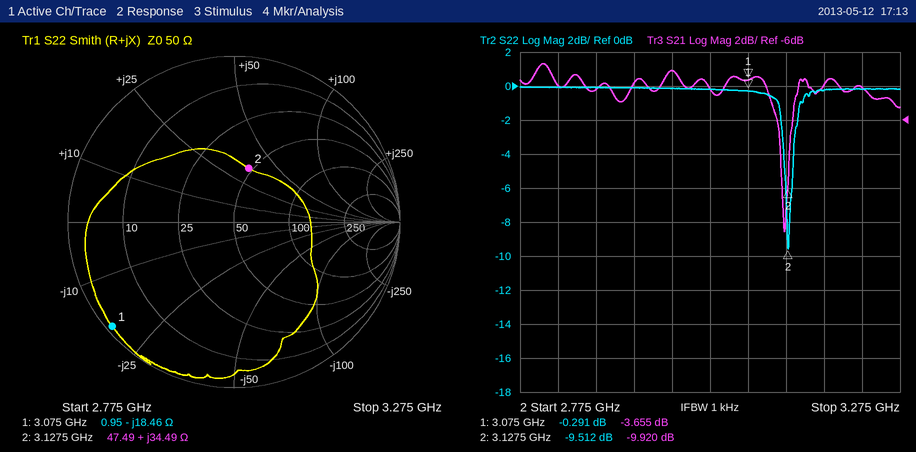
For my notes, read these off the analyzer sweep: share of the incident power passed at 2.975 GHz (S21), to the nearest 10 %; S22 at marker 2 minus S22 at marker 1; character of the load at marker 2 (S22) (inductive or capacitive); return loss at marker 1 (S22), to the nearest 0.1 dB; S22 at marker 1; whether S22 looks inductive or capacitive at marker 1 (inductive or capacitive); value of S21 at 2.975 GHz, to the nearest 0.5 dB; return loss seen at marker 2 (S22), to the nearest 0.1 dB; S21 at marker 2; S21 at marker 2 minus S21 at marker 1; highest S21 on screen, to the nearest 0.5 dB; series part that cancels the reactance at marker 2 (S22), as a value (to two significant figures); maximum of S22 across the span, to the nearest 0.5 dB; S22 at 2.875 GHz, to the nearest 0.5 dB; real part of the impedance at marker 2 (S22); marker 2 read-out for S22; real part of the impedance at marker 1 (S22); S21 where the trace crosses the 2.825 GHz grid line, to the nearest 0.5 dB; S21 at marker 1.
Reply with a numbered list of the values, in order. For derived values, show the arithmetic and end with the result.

1. 10^(-3/10) ≈ 50 %
2. -9.512 − (-0.291) = -9.221 dB
3. inductive
4. 0.3 dB
5. -0.291 dB
6. capacitive
7. -3.0 dB
8. 9.5 dB
9. -9.920 dB
10. -9.92 − (-3.655) = -6.265 dB
11. -2.5 dB
12. C = 1/(2π × 3.1275 GHz × 34.49 Ω) ≈ 1.5 pF
13. 0.0 dB
14. 0.0 dB
15. 47.49 Ω
16. -9.512 dB
17. 0.95 Ω
18. -4.0 dB
19. -3.655 dB
